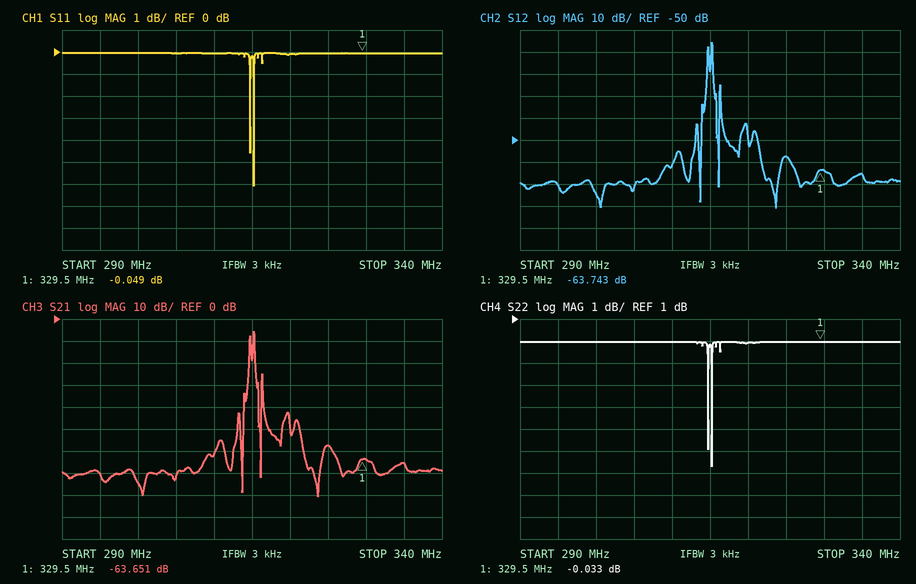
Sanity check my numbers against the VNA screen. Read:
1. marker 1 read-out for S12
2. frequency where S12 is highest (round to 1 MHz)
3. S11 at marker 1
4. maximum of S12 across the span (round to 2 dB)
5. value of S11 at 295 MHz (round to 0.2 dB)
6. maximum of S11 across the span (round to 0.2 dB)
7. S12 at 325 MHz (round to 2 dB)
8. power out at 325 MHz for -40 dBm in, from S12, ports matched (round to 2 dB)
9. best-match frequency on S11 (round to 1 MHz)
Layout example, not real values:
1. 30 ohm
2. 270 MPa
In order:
1. -63.743 dB
2. 315 MHz
3. -0.049 dB
4. -6 dB
5. 0.0 dB
6. 0.0 dB
7. -58 dB
8. -98 dBm
9. 315 MHz
